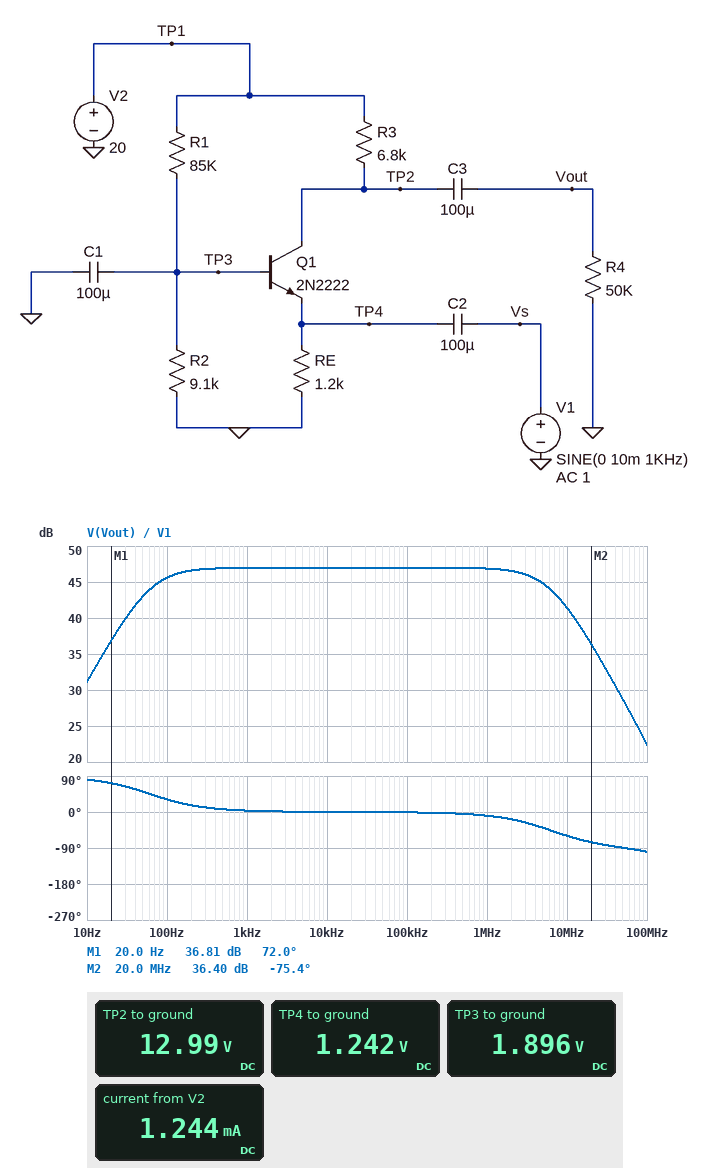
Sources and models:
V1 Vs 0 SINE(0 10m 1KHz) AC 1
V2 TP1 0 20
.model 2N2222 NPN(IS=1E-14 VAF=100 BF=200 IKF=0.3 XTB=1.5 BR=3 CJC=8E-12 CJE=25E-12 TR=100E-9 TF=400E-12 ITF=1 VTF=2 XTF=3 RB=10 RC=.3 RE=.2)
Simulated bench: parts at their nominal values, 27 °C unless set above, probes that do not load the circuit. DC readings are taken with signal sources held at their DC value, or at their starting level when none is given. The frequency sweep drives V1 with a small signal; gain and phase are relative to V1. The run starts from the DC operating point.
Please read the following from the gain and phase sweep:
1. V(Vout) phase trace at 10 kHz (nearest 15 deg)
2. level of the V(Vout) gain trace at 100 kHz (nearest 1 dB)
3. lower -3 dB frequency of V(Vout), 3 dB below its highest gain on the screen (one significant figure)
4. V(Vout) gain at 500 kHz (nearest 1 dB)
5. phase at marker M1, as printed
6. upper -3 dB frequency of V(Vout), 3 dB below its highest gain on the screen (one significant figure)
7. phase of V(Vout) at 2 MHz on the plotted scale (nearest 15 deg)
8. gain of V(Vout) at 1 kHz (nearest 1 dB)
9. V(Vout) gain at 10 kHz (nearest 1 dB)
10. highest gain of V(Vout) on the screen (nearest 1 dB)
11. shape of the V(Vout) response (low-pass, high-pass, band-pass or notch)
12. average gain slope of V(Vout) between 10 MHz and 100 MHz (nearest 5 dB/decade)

0 deg
47 dB
60 Hz
47 dB
72.0 deg
6 MHz
-15 deg
47 dB
47 dB
47 dB
band-pass
-20 dB/decade
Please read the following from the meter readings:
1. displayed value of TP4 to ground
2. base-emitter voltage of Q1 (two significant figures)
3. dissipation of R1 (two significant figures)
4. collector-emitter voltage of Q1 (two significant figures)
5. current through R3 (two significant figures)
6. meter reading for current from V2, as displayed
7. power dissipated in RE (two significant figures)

1.242 V
650 mV
3.9 mW
12 V
1.0 mA
1.244 mA
1.3 mW
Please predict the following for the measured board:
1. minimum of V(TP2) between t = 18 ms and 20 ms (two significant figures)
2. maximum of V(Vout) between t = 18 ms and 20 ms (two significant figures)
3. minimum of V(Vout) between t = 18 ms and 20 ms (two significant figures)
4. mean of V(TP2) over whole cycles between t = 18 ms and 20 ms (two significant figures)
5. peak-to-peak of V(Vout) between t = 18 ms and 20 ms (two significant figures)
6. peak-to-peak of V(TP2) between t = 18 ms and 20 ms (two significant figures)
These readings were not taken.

11 V
2.0 V
-2.4 V
13 V
4.4 V
4.4 V
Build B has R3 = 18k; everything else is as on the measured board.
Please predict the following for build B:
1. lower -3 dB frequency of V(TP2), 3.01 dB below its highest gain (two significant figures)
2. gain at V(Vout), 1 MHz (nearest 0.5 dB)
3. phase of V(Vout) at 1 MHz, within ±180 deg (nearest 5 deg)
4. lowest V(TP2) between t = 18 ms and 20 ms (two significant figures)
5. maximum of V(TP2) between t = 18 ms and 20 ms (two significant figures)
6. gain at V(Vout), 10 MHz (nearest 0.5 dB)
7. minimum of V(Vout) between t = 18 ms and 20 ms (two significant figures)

57 Hz
50.0 dB
-45 deg
1.3 V
5.2 V
33.0 dB
-310 mV
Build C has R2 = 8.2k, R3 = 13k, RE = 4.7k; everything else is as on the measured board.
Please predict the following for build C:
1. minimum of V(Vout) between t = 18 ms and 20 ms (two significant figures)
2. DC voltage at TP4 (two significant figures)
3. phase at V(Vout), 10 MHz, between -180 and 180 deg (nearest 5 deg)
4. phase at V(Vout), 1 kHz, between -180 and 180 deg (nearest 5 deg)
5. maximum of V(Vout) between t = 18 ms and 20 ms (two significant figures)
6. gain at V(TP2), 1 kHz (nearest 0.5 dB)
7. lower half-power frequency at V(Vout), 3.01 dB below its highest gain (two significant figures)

-1.0 V
1.1 V
-65 deg
0 deg
830 mV
39.5 dB
15 Hz
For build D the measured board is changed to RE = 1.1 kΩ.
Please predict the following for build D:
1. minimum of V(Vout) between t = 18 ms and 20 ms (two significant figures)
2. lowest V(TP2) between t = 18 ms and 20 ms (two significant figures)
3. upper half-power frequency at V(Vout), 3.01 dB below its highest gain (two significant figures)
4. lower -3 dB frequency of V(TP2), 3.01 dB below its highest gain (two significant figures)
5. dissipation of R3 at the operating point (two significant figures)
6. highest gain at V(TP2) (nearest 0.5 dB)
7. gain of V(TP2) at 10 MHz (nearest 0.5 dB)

-2.6 V
9.8 V
6.0 MHz
66 Hz
8.5 mW
47.5 dB
42.0 dB
